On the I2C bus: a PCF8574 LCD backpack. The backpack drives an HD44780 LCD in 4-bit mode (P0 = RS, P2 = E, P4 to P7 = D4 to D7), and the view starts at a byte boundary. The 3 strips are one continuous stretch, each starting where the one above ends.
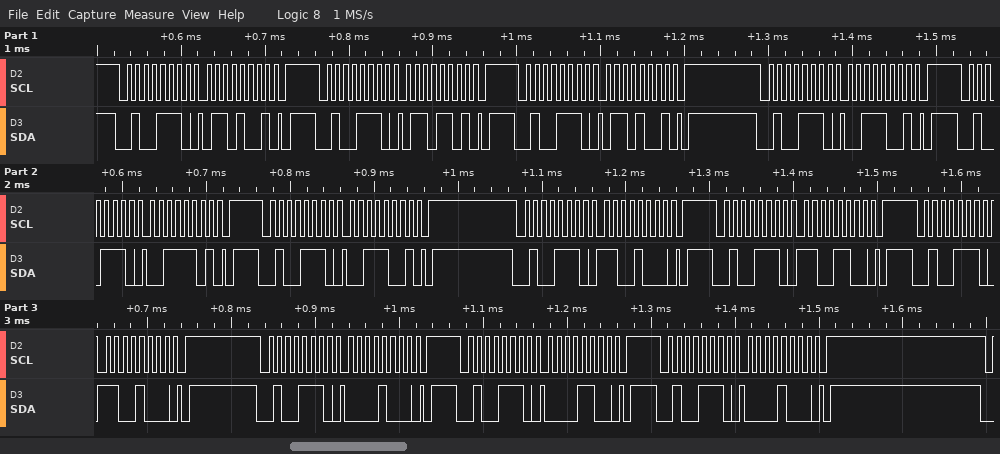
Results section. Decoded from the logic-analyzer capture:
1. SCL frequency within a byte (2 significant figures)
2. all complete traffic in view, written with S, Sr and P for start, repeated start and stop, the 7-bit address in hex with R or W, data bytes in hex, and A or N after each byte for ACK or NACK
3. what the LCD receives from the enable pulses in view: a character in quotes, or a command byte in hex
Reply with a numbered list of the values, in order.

1. 100 kHz
2. S 27W A 69 A P S 27W A 6D A P S 27W A 69 A P S 27W A 39 A P S 27W A 3D A P S 27W A 39 A P S 27W A C8 A P S 27W A CC A P S 27W A C8 A P S 27W A 08 A P S 27W A 0C A P S 27W A 08 A P
3. 'c' 0xC0
